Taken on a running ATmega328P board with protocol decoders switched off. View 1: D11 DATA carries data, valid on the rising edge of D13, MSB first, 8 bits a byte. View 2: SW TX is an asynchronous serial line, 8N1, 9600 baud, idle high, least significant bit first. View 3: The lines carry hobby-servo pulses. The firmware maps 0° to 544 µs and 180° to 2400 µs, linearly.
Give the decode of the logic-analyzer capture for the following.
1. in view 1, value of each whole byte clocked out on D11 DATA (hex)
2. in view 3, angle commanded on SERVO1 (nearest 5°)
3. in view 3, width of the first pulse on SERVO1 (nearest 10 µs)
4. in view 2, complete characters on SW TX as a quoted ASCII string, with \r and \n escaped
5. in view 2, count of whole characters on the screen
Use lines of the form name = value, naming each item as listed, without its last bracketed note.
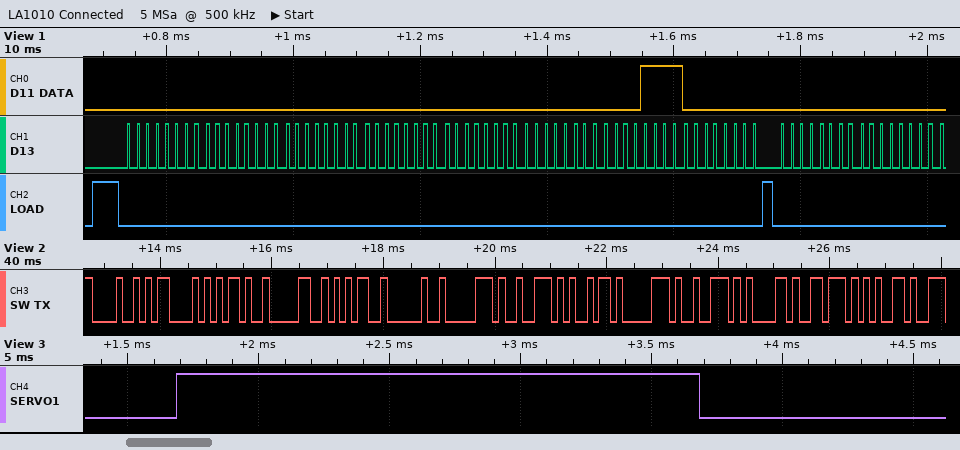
in view 1, value of each whole byte clocked out on D11 DATA = 00 00 00 00 00 00 0F 00 00 00
in view 3, angle commanded on SERVO1 = 140°
in view 3, width of the first pulse on SERVO1 = 2000 µs
in view 2, complete characters on SW TX as a quoted ASCII string, with \r and \n escaped = "HC-05 priprave"
in view 2, count of whole characters on the screen = 14
